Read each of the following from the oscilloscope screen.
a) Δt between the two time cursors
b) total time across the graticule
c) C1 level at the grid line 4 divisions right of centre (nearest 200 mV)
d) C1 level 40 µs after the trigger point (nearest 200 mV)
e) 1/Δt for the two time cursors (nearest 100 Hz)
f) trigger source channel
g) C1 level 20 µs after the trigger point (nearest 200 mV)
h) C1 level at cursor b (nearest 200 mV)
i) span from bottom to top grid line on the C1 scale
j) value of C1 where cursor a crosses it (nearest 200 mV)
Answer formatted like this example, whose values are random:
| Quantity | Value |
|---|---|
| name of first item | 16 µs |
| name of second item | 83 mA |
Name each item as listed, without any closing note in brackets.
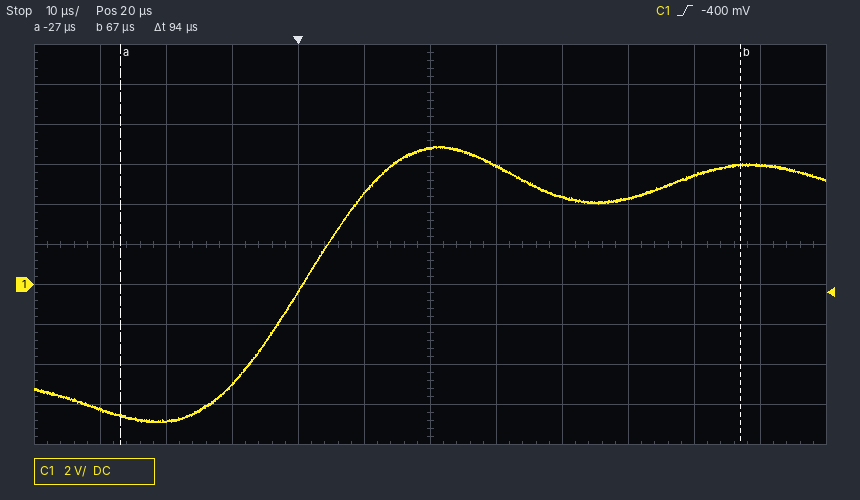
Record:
| Quantity | Value |
|---|---|
| Δt between the two time cursors | 94 µs |
| total time across the graticule | 120 µs |
| C1 level at the grid line 4 divisions right of centre | 5.4 V |
| C1 level 40 µs after the trigger point | 4.4 V |
| 1/Δt for the two time cursors | 10.6 kHz |
| trigger source channel | C1 |
| C1 level 20 µs after the trigger point | 6.8 V |
| C1 level at cursor b | 6.0 V |
| span from bottom to top grid line on the C1 scale | 20 V |
| value of C1 where cursor a crosses it | -6.6 V |
